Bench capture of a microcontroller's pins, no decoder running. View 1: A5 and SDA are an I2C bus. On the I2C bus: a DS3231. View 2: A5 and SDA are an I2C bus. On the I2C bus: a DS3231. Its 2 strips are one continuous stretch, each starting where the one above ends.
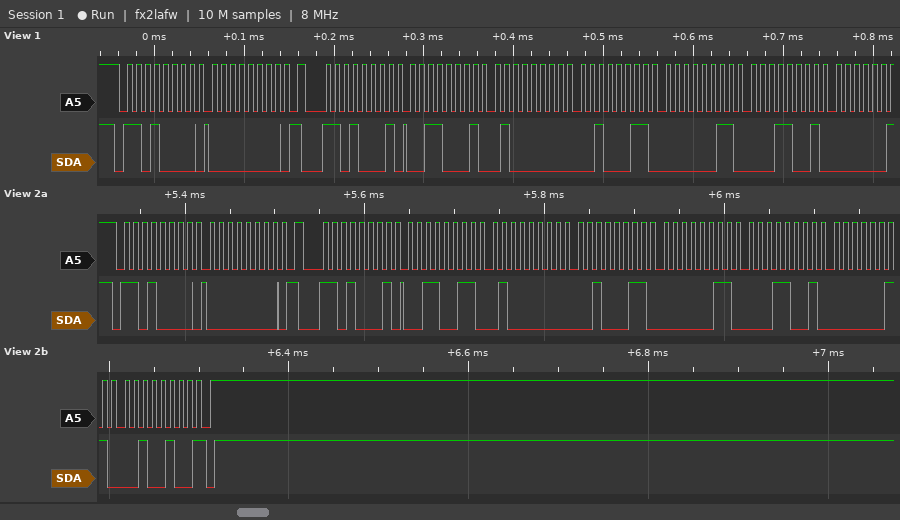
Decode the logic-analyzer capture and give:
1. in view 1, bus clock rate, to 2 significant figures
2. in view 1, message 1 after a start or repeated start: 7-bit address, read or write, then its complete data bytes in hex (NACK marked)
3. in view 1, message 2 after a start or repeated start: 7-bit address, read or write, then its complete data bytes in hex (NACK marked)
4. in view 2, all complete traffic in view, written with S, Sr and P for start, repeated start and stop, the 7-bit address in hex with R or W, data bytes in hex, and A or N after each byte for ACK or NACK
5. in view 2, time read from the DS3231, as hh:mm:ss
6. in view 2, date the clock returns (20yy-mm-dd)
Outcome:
100 kHz
0x68 write: 00
0x68 read: 31 40 23 03 19
S 68W A 00 A Sr 68R A 33 A 40 A 23 A 03 A 19 A 03 A 24 N P
23:40:33
2024-03-19
